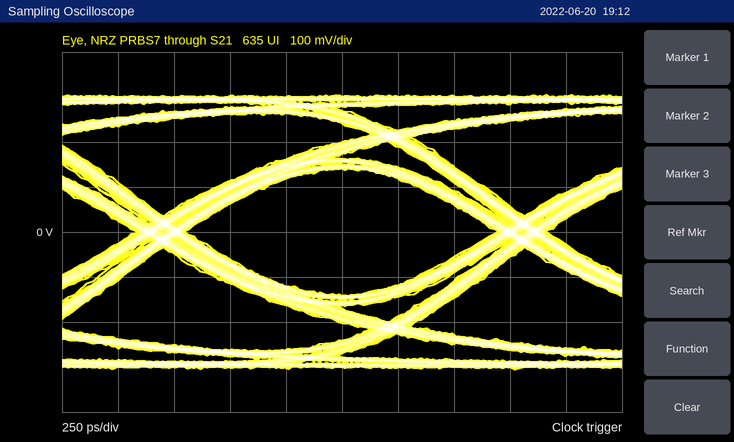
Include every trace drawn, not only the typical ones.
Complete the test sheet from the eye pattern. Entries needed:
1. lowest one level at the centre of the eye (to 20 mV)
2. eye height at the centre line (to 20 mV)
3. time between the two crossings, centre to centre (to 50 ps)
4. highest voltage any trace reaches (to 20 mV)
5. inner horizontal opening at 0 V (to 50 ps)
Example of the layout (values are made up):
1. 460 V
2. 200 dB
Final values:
1. 140 mV
2. 280 mV
3. 1.60 ns
4. 300 mV
5. 1.40 ns
